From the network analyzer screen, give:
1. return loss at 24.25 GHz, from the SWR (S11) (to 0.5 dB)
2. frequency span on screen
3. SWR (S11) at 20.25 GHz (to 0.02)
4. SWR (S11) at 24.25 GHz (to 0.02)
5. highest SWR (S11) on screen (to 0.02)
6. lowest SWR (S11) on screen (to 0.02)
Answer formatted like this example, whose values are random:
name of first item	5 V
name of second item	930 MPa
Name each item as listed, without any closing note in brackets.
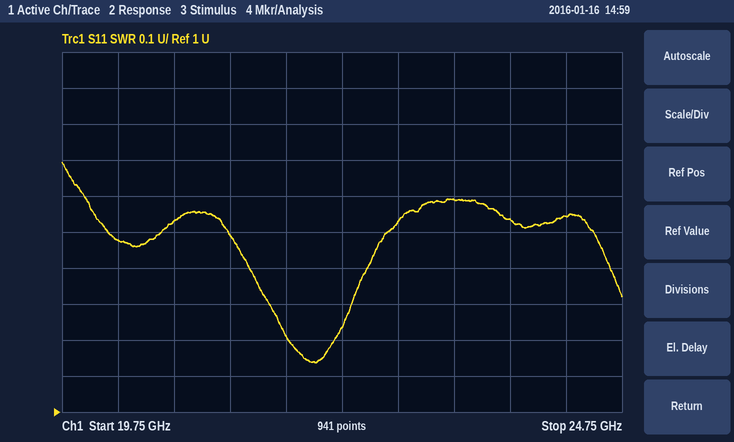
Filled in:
return loss at 24.25 GHz, from the SWR (S11)	13.5 dB
frequency span on screen	5 GHz
SWR (S11) at 20.25 GHz	1.48
SWR (S11) at 24.25 GHz	1.54
highest SWR (S11) on screen	1.70
lowest SWR (S11) on screen	1.14
